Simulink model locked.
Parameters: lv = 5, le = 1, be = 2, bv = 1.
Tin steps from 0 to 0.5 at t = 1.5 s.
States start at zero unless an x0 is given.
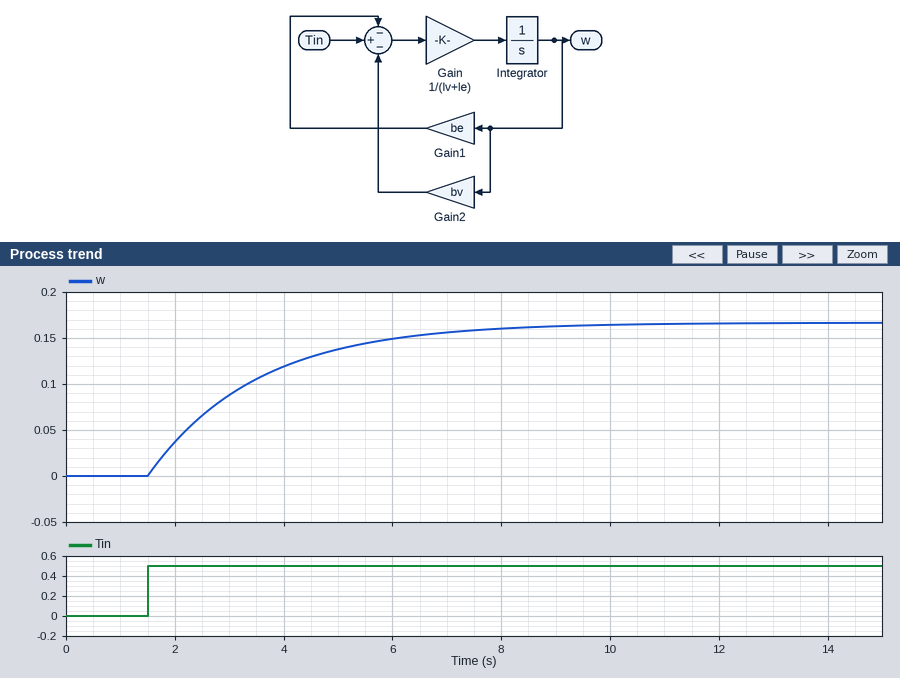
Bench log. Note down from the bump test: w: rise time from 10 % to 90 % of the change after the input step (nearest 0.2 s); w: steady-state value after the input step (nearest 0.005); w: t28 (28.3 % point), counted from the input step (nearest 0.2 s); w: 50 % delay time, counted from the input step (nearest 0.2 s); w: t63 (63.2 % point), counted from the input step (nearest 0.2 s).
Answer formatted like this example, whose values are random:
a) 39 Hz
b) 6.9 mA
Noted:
a) 4.4 s
b) 0.165
c) 0.6 s
d) 1.4 s
e) 2.0 s
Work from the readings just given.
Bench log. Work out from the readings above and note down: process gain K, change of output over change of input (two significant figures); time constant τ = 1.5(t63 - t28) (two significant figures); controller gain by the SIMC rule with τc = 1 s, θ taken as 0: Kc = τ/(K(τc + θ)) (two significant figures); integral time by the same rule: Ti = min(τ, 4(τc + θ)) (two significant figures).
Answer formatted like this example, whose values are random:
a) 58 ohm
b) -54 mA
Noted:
a) 0.33
b) 2.1 s
c) 6.4
d) 2.1 s
